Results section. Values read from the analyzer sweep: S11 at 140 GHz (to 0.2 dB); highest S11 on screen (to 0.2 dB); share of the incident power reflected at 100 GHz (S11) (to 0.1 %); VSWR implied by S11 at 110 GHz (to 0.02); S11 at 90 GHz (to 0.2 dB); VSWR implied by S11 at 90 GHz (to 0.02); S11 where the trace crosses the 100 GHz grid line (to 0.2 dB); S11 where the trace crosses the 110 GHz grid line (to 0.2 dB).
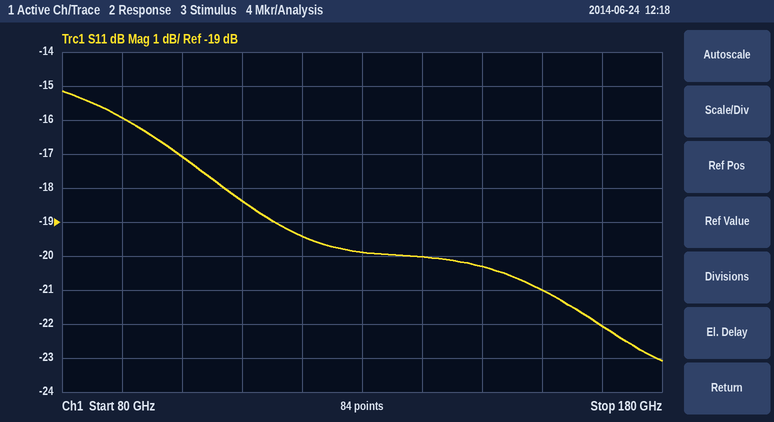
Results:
-20.0 dB
-15.2 dB
2.0 %
1.28
-16.0 dB
1.38
-17.0 dB
-18.4 dB
